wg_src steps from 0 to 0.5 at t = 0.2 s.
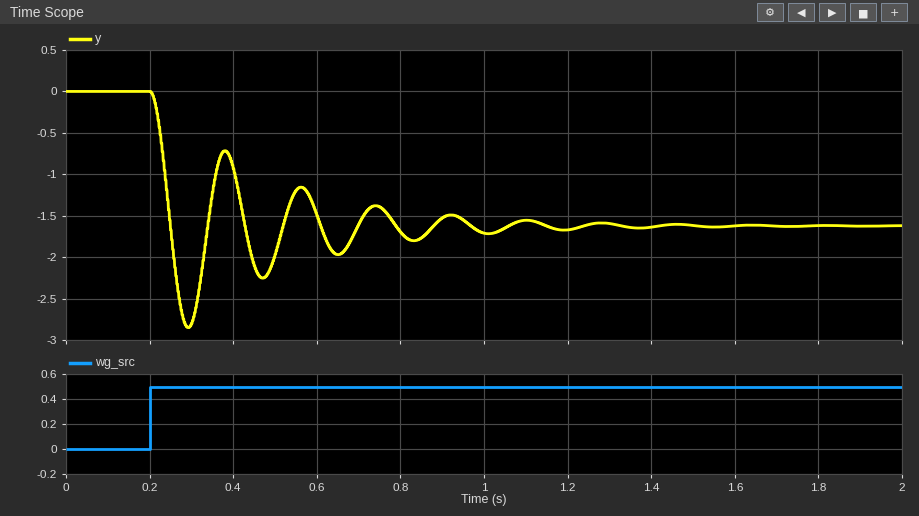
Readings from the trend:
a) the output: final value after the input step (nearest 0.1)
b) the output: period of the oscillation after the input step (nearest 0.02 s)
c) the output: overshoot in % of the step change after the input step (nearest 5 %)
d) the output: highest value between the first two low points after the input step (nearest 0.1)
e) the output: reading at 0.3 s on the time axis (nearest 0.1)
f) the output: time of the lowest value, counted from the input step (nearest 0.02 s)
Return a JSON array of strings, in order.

["-1.6", "0.18 s", "75 %", "-0.7", "-2.8", "0.10 s"]
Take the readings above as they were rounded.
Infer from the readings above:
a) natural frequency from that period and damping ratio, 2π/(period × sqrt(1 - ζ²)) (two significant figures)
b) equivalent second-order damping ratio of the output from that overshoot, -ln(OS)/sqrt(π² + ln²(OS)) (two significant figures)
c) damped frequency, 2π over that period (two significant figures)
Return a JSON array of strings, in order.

["35 rad/s", "0.091", "35 rad/s"]
